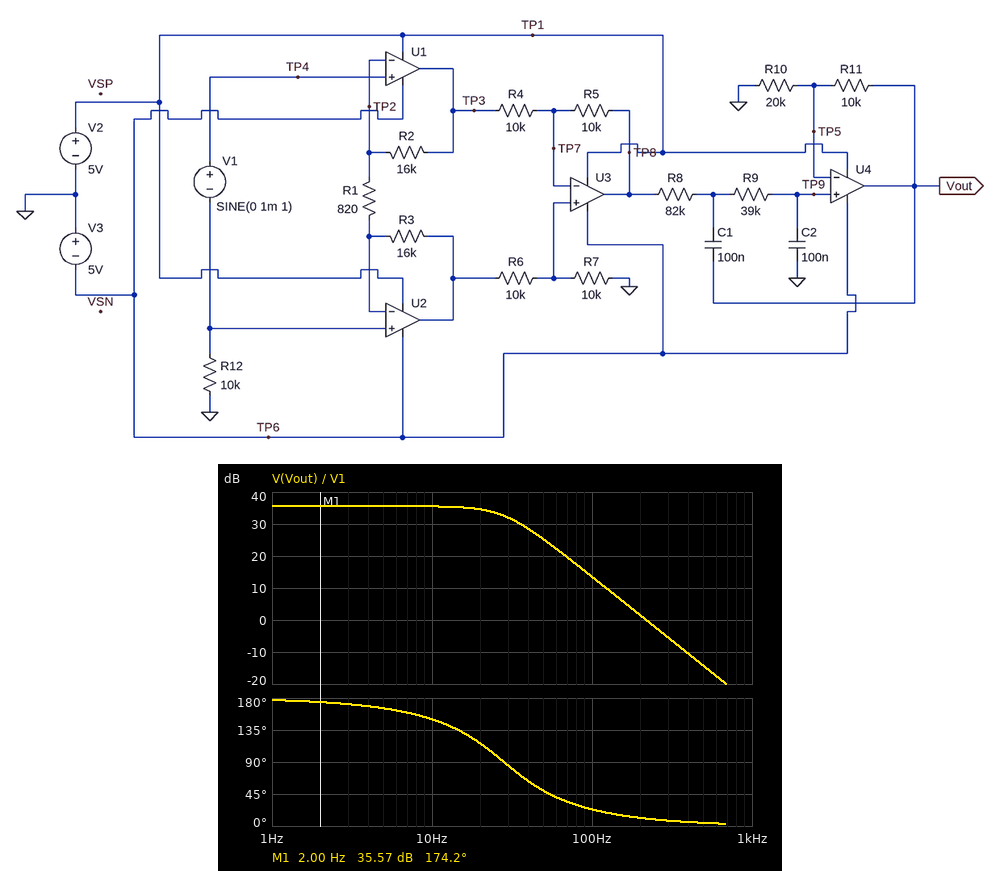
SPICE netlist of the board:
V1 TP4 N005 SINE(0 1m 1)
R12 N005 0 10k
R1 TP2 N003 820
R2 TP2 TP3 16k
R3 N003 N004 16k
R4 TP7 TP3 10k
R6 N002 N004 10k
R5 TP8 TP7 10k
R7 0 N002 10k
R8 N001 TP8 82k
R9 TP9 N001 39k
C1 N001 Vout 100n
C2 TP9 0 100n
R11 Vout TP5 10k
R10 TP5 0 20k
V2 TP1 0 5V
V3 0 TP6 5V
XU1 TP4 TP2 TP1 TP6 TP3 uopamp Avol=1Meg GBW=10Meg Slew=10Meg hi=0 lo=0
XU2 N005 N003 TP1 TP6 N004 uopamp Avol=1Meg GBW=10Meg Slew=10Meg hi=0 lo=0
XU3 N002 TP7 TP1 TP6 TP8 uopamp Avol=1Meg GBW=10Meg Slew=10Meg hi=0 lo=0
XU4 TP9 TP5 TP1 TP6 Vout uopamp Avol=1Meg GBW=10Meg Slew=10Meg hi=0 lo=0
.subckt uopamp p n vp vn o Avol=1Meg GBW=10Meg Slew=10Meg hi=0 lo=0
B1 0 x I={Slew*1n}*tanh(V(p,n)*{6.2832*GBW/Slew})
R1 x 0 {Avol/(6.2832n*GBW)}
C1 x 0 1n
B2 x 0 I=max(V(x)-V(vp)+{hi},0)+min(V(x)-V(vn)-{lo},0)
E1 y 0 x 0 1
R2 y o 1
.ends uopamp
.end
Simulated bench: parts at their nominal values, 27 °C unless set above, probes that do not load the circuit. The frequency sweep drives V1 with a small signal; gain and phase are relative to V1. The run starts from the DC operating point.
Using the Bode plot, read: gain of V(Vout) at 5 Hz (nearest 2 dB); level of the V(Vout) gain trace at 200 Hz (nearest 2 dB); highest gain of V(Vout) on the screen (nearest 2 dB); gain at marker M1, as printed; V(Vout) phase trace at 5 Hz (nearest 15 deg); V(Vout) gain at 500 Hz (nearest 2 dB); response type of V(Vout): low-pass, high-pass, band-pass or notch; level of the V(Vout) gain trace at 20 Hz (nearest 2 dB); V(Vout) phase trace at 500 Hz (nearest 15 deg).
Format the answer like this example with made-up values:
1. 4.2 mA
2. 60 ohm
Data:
1. 36 dB
2. 2 dB
3. 36 dB
4. 35.57 dB
5. 165 deg
6. -14 dB
7. low-pass
8. 34 dB
9. 0 deg
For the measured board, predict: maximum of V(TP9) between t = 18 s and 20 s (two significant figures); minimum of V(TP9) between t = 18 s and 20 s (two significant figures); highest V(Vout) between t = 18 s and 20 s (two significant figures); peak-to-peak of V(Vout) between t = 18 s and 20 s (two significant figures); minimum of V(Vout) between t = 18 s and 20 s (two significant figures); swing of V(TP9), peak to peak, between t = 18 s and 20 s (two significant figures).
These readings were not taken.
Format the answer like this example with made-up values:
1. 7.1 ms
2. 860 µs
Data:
1. 40 mV
2. -40 mV
3. 60 mV
4. 120 mV
5. -60 mV
6. 80 mV
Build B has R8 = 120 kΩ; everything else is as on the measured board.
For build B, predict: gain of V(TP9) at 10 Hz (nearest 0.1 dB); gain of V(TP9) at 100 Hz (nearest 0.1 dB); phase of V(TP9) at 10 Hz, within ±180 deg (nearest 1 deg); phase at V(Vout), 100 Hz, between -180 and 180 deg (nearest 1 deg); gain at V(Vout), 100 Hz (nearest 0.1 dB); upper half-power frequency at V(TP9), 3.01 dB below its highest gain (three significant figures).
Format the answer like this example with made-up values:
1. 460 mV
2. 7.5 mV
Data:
1. 31.8 dB
2. 6.7 dB
3. 143 deg
4. 20 deg
5. 10.2 dB
6. 22.7 Hz
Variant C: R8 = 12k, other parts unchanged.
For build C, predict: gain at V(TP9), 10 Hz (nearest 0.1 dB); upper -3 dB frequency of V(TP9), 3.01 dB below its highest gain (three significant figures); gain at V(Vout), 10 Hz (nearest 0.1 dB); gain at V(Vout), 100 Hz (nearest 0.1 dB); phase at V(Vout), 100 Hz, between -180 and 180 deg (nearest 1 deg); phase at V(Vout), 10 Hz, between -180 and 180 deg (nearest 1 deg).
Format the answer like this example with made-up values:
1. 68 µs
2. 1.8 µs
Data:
1. 31.9 dB
2. 44.8 Hz
3. 35.4 dB
4. 26.2 dB
5. 73 deg
6. 164 deg
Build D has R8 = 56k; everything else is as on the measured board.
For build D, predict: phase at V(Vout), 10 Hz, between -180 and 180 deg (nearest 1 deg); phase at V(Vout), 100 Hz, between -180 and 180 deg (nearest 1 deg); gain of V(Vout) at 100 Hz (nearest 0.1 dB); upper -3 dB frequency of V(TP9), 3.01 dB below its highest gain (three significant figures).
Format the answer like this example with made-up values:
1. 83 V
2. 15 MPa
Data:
1. 155 deg
2. 29 deg
3. 16.8 dB
4. 33.6 Hz
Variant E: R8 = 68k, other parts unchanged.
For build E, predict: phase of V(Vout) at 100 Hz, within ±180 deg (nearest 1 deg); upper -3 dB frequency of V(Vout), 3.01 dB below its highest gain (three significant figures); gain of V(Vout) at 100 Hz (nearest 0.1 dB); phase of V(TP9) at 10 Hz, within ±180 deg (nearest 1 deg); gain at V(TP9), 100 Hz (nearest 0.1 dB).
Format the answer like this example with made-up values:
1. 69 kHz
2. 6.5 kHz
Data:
1. 26 deg
2. 30.8 Hz
3. 15.1 dB
4. 153 deg
5. 11.6 dB
